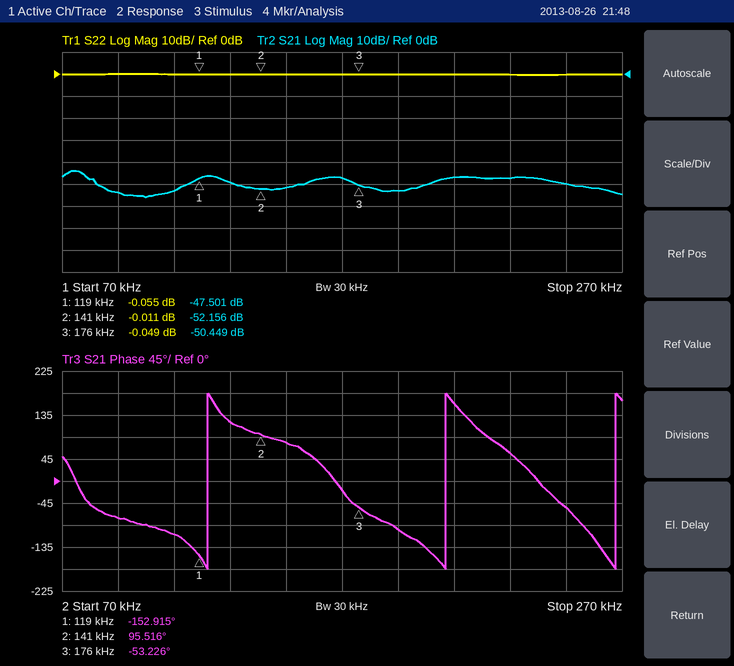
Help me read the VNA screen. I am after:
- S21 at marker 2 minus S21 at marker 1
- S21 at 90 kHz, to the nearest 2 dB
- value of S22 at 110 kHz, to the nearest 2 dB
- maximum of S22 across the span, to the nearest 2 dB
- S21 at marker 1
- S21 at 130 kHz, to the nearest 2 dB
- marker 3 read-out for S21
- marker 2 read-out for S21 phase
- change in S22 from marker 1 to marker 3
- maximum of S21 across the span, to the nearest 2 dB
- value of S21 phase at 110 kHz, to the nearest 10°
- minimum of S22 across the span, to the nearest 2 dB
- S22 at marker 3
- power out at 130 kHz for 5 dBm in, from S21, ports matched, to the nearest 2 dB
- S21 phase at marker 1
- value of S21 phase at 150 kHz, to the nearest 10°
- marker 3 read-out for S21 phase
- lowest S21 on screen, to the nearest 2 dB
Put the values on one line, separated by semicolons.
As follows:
-4.655 dB; -54 dB; 0 dB; 0 dB; -47.501 dB; -50 dB; -50.449 dB; 95.516°; 0.006 dB; -44 dB; -110°; 0 dB; -0.049 dB; -44 dBm; -152.915°; 80°; -53.226°; -56 dB
